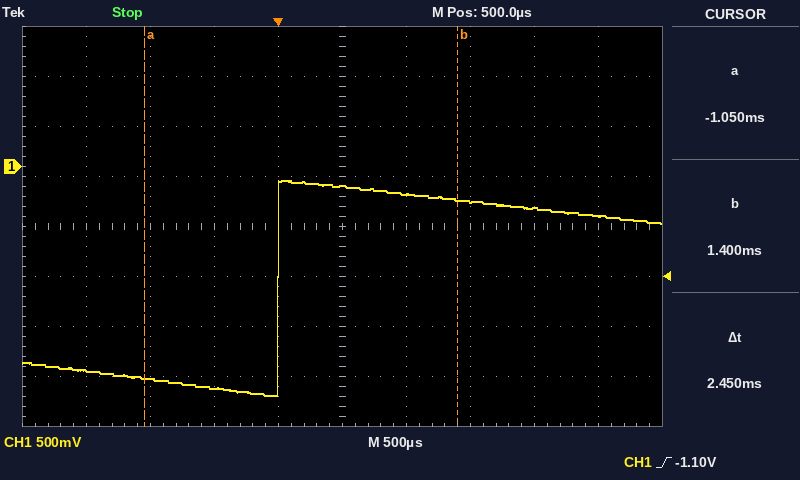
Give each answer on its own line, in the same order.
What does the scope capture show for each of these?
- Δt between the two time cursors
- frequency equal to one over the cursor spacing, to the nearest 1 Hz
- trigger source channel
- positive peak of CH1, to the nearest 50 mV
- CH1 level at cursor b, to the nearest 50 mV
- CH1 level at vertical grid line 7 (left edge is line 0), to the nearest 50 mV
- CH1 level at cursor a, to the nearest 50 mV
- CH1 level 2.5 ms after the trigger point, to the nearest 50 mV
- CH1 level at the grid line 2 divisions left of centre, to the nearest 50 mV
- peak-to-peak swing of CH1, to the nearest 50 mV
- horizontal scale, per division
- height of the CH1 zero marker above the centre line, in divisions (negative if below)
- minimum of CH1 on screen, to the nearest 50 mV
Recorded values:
2.45 ms
408 Hz
CH1
-150 mV
-350 mV
-350 mV
-2.10 V
-500 mV
-2.20 V
2.15 V
500 µs
+1.2 div
-2.30 V
